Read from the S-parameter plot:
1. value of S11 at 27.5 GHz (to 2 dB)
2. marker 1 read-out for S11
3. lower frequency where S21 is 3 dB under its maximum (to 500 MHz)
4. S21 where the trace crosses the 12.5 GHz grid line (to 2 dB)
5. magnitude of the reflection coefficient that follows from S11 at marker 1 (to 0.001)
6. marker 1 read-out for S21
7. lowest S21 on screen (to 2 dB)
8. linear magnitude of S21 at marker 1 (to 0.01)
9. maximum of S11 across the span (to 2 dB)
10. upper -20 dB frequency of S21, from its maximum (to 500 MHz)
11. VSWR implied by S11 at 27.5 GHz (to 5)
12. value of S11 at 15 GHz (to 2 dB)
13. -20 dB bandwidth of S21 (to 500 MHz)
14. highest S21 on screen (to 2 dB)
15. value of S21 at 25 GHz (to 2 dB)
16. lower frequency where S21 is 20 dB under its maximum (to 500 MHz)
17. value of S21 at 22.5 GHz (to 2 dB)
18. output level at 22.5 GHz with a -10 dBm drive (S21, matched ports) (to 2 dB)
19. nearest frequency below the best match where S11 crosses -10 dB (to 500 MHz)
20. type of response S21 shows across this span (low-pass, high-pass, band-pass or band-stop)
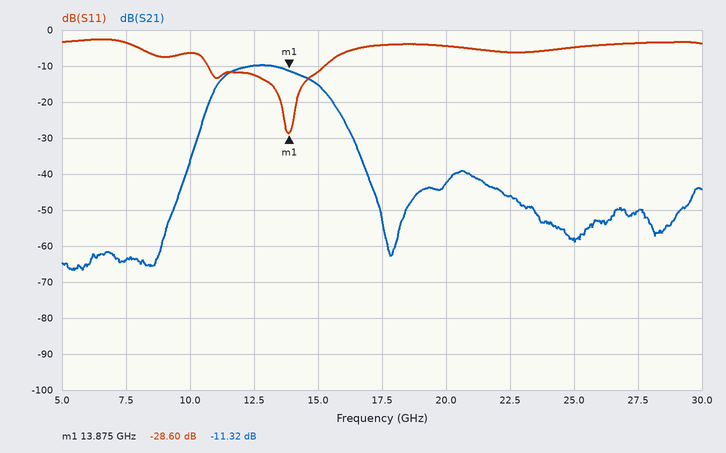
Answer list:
-4 dB
-28.60 dB
11.5 GHz
-10 dB
0.037
-11.32 dB
-66 dB
0.27
-2 dB
16.5 GHz
5
-12 dB
6.0 GHz
-10 dB
-58 dB
10.5 GHz
-46 dB
-56 dBm
10.5 GHz
band-pass
